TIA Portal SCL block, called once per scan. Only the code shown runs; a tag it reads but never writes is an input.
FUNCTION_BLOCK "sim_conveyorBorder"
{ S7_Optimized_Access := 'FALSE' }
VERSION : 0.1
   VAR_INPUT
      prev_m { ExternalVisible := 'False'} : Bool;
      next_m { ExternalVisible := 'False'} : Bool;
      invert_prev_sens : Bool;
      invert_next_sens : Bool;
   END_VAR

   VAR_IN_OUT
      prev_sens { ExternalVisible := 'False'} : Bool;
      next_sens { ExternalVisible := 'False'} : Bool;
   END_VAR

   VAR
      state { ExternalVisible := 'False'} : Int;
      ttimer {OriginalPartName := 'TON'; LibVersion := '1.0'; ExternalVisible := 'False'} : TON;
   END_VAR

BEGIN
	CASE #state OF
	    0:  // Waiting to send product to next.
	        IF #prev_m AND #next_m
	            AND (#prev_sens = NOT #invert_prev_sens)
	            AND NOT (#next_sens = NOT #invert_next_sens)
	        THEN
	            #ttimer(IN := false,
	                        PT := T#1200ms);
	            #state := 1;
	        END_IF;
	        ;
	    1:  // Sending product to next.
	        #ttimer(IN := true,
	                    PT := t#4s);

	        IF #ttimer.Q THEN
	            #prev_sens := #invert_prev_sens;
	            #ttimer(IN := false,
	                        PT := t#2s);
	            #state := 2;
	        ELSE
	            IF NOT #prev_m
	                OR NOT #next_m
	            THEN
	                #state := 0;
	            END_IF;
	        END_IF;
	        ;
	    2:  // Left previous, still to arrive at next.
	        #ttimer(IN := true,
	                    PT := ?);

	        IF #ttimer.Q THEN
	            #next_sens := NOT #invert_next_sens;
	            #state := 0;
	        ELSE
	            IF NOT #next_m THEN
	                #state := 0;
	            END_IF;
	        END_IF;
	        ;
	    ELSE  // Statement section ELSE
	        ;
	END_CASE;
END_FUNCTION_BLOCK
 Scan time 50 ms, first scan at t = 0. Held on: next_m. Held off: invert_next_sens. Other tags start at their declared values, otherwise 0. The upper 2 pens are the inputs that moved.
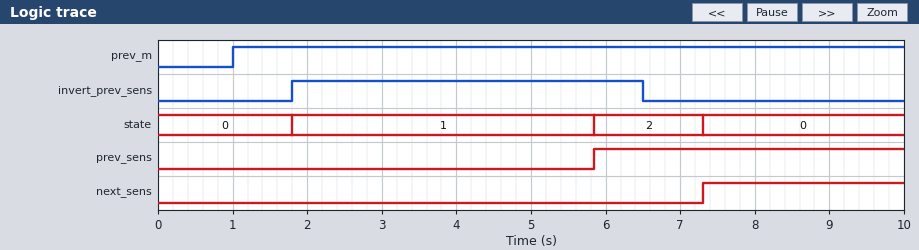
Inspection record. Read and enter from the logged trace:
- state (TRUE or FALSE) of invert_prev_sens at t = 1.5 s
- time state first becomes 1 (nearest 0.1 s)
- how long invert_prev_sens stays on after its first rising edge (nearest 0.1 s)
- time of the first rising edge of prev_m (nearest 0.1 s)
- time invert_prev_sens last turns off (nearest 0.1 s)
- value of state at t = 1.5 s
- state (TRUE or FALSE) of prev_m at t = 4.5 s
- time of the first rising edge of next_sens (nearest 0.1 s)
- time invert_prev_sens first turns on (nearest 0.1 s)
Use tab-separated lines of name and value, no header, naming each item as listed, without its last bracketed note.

state (TRUE or FALSE) of invert_prev_sens at t = 1.5 s	FALSE
time state first becomes 1	1.8 s
how long invert_prev_sens stays on after its first rising edge	4.7 s
time of the first rising edge of prev_m	1.0 s
time invert_prev_sens last turns off	6.5 s
value of state at t = 1.5 s	0
state (TRUE or FALSE) of prev_m at t = 4.5 s	TRUE
time of the first rising edge of next_sens	7.3 s
time invert_prev_sens first turns on	1.8 s
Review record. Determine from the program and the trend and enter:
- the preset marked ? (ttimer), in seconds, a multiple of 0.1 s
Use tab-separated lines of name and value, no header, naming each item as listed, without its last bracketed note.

the preset marked ? (ttimer), in seconds, a multiple of 0.1 s	1.4 s
